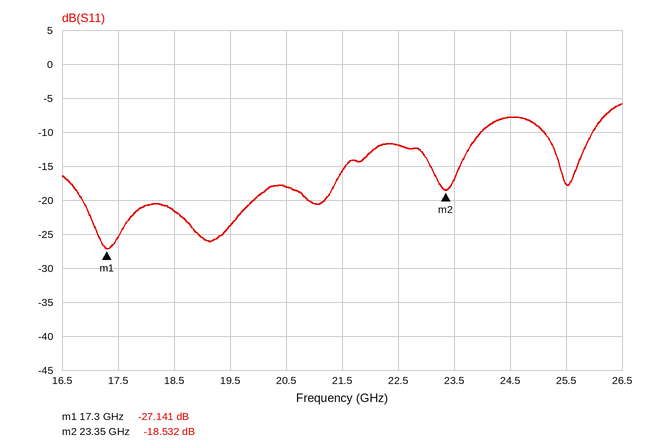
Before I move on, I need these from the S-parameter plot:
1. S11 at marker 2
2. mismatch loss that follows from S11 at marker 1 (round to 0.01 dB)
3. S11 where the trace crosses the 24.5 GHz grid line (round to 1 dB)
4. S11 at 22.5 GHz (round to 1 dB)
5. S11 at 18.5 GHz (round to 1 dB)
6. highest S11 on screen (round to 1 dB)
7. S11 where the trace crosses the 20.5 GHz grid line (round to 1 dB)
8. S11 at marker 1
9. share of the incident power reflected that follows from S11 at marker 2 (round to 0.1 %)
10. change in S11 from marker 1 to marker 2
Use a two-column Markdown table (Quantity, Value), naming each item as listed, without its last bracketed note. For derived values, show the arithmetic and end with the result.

| Quantity | Value |
|---|---|
| S11 at marker 2 | -18.532 dB |
| mismatch loss that follows from S11 at marker 1 | −10 log10(1 − 10^(-27.141/10)) ≈ 0.01 dB |
| S11 where the trace crosses the 24.5 GHz grid line | -8 dB |
| S11 at 22.5 GHz | -12 dB |
| S11 at 18.5 GHz | -22 dB |
| highest S11 on screen | -6 dB |
| S11 where the trace crosses the 20.5 GHz grid line | -18 dB |
| S11 at marker 1 | -27.141 dB |
| share of the incident power reflected that follows from S11 at marker 2 | 10^(-18.532/10) ≈ 1.4 % |
| change in S11 from marker 1 to marker 2 | -18.532 − (-27.141) = 8.609 dB |
